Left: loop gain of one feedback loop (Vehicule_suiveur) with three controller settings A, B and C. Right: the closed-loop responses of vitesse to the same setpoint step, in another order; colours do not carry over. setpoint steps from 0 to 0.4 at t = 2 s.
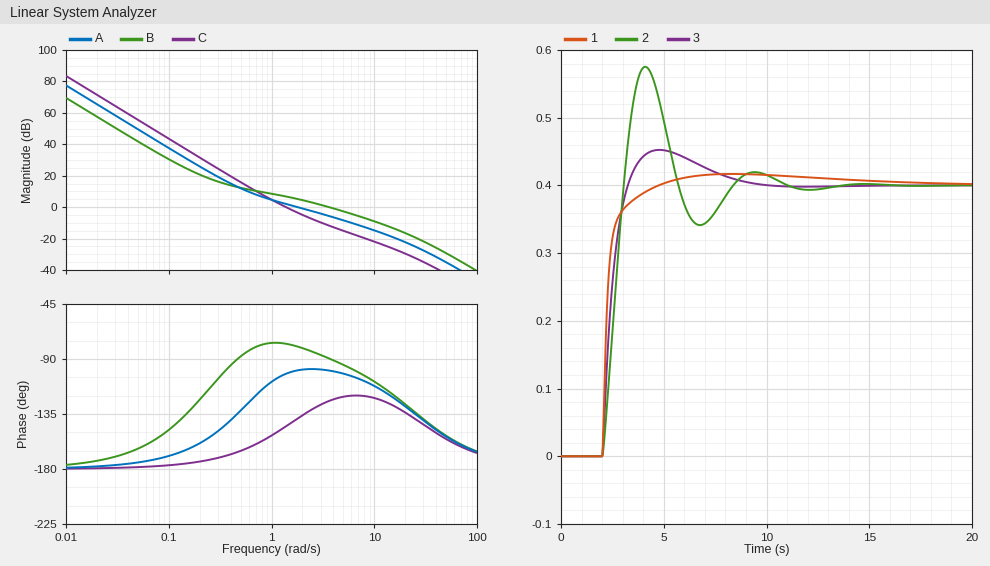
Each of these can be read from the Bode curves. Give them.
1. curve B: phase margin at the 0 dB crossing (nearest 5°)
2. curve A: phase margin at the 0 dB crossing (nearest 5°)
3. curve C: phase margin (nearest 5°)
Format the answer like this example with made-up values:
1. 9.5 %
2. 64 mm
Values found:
1. 90°
2. 80°
3. 35°
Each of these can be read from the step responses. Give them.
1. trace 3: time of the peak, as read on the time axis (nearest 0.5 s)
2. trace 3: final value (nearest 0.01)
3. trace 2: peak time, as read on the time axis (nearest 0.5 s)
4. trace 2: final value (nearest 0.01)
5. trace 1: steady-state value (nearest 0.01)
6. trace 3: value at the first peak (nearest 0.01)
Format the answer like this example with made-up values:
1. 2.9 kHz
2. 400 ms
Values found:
1. 5.0 s
2. 0.40
3. 4.0 s
4. 0.40
5. 0.40
6. 0.45
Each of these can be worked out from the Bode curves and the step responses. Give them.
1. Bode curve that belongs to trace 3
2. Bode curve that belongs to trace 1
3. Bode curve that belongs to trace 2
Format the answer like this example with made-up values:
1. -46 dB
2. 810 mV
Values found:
1. A
2. B
3. C
